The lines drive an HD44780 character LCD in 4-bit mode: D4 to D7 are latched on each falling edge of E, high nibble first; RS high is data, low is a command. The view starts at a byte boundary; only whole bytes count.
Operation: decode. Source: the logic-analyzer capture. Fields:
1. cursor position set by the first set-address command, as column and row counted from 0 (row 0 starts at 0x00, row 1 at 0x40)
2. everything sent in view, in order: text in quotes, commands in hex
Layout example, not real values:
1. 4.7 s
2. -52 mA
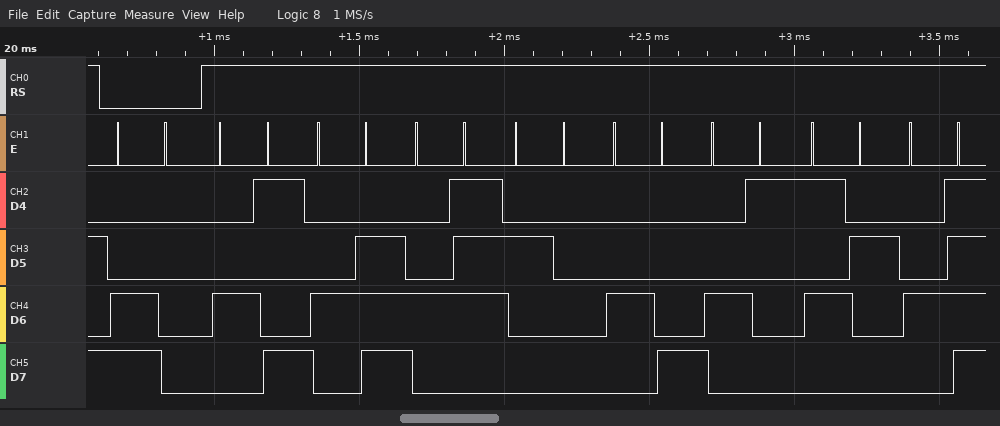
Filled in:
1. column 0, row 1
2. 0xC0 "ING HARO"
